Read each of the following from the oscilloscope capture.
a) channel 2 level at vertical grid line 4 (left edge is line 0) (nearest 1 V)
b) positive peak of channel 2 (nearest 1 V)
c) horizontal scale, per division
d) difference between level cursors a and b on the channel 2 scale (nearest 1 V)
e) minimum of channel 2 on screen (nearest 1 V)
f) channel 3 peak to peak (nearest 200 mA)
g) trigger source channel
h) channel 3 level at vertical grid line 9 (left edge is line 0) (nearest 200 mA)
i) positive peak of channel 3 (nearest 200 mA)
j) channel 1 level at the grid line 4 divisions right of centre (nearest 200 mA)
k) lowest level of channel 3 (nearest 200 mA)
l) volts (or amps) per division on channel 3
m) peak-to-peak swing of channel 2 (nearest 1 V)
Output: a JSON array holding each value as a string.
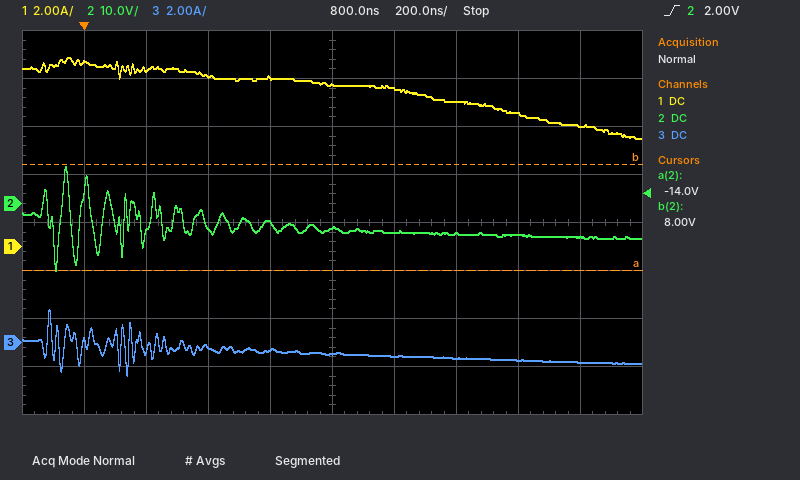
["-4 V", "8 V", "200 ns", "22 V", "-14 V", "2.8 A", "channel 2", "-800 mA", "1.4 A", "5.0 A", "-1.4 A", "2 A", "22 V"]
